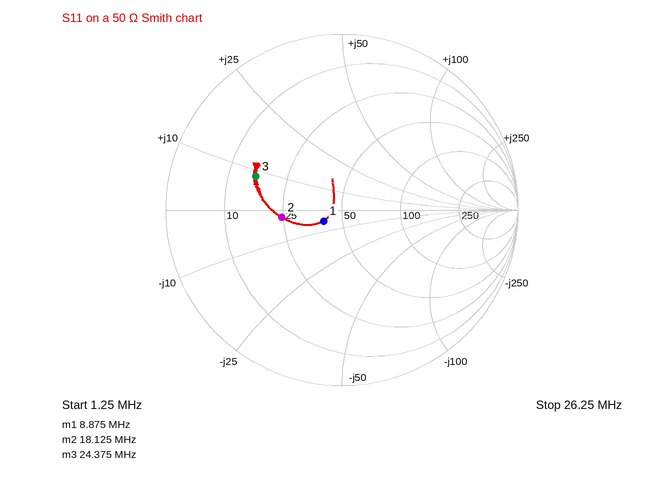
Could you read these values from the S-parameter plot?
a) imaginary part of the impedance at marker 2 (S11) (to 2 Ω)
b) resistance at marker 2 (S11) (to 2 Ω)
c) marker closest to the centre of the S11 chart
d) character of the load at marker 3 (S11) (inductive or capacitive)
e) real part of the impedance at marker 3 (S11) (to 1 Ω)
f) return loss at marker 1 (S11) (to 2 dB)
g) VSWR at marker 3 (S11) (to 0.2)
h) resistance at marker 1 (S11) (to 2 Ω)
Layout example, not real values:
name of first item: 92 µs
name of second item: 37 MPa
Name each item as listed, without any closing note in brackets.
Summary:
imaginary part of the impedance at marker 2 (S11): -2 Ω
resistance at marker 2 (S11): 24 Ω
marker closest to the centre of the S11 chart: marker 1
character of the load at marker 3 (S11): inductive
real part of the impedance at marker 3 (S11): 16 Ω
return loss at marker 1 (S11): 18 dB
VSWR at marker 3 (S11): 3.2
resistance at marker 1 (S11): 40 Ω
